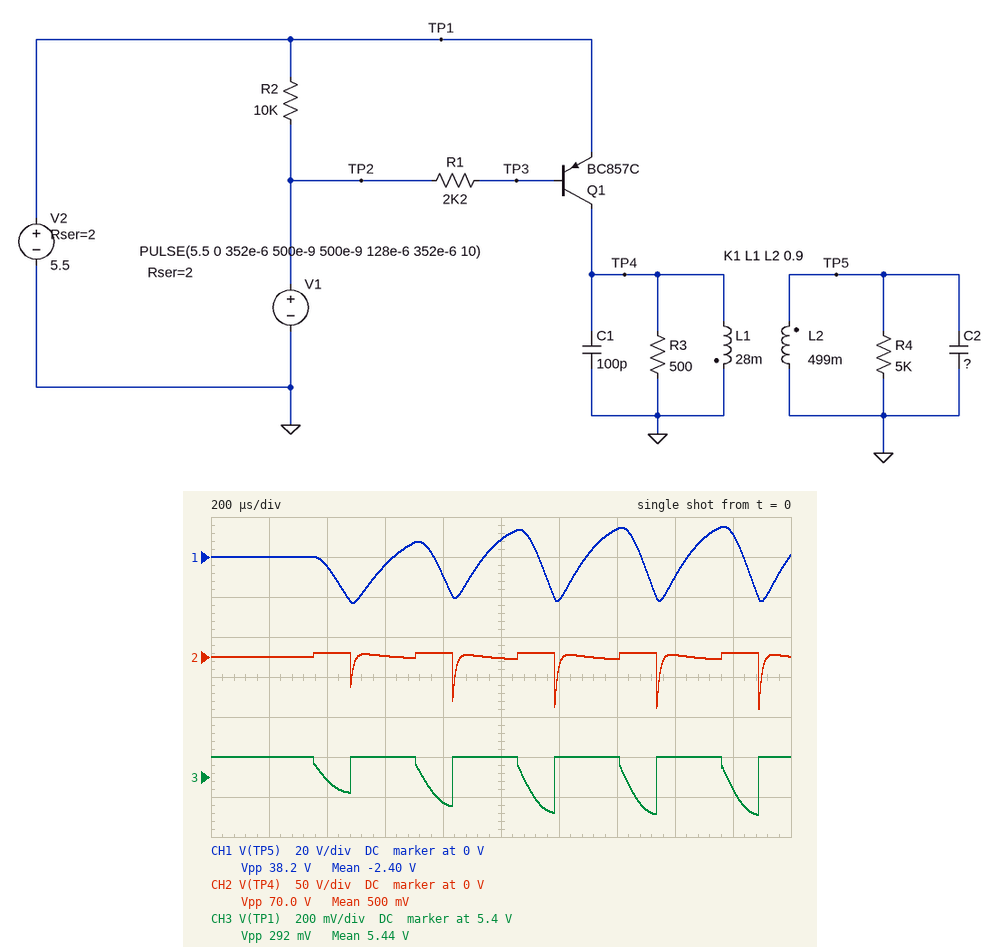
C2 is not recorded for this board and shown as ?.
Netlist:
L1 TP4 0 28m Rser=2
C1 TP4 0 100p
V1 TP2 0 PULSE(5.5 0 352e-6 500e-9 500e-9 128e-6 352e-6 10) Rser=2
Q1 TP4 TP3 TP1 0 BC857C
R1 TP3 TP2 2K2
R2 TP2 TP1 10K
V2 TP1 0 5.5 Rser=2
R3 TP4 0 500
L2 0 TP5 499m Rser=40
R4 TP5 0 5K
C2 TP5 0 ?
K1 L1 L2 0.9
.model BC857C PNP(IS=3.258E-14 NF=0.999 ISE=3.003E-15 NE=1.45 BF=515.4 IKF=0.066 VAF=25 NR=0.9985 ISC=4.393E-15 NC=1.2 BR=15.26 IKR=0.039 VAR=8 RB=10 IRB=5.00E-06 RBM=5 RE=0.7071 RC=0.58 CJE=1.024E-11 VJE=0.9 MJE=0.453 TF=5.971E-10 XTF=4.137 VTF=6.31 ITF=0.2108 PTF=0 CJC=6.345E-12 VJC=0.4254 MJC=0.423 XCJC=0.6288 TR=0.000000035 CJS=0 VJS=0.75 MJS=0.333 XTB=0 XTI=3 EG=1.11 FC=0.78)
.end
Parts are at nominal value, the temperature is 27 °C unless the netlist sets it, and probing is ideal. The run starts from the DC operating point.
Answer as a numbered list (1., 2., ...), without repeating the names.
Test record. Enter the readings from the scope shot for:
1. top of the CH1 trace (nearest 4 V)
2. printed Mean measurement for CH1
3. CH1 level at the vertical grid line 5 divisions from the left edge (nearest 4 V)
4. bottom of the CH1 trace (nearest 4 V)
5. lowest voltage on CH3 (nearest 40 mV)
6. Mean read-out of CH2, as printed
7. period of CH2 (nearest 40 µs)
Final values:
1. 16 V
2. -2.40 V
3. 8 V
4. -24 V
5. 5.20 V
6. 500 mV
7. 360 µs
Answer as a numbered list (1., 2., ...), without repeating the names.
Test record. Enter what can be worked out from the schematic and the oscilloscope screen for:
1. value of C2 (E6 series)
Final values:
1. 47 nF
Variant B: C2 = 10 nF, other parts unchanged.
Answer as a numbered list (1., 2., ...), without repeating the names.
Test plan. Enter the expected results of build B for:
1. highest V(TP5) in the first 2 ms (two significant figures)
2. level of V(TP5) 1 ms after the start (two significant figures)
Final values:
1. 18 V
2. 13 V
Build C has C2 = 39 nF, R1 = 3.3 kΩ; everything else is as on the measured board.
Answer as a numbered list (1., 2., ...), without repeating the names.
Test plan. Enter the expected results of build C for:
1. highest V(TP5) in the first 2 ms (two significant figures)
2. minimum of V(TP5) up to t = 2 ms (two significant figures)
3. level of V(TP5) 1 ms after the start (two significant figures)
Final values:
1. 18 V
2. -27 V
3. 11 V
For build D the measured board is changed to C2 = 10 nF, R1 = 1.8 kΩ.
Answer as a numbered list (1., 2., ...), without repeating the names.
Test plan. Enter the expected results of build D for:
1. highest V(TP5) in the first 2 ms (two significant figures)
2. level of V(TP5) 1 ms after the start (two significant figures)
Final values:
1. 18 V
2. 13 V
